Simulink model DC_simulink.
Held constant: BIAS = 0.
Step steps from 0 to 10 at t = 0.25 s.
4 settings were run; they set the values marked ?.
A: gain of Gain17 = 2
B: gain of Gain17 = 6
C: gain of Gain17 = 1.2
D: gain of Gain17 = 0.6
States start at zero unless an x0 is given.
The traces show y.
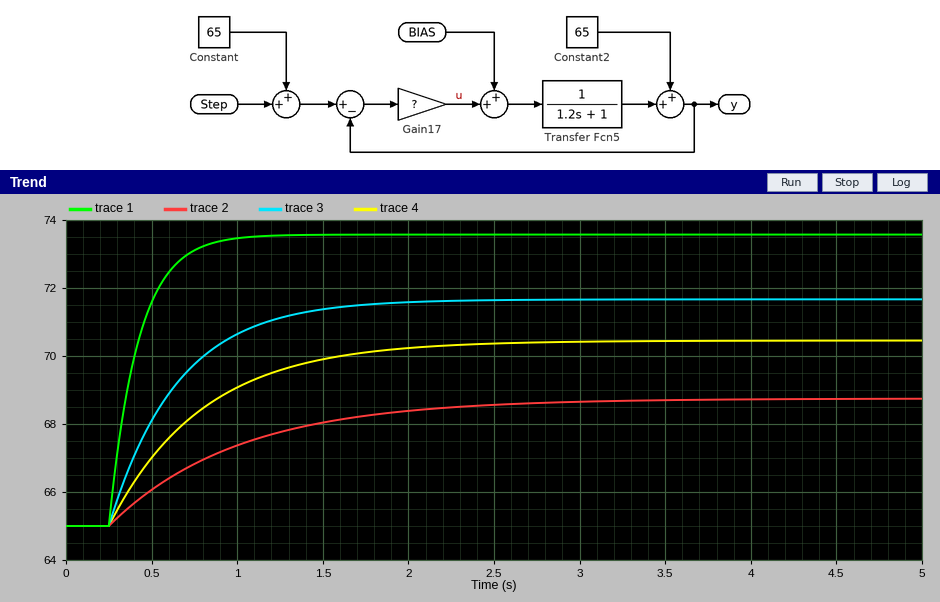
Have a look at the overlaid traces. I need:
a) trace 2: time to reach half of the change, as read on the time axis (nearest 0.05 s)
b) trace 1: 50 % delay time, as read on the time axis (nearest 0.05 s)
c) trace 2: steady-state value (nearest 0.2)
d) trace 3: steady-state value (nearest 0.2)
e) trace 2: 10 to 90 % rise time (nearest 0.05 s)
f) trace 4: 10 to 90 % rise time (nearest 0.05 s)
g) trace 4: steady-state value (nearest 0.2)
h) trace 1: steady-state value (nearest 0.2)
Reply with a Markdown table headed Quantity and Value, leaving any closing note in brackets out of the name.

| Quantity | Value |
|---|---|
| trace 2: time to reach half of the change, as read on the time axis | 0.75 s |
| trace 1: 50 % delay time, as read on the time axis | 0.35 s |
| trace 2: steady-state value | 68.8 |
| trace 3: steady-state value | 71.6 |
| trace 2: 10 to 90 % rise time | 1.65 s |
| trace 4: 10 to 90 % rise time | 1.20 s |
| trace 4: steady-state value | 70.4 |
| trace 1: steady-state value | 73.6 |
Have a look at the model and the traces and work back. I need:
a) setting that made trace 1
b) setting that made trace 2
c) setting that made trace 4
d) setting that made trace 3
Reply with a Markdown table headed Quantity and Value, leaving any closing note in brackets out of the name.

| Quantity | Value |
|---|---|
| setting that made trace 1 | B |
| setting that made trace 2 | D |
| setting that made trace 4 | C |
| setting that made trace 3 | A |
